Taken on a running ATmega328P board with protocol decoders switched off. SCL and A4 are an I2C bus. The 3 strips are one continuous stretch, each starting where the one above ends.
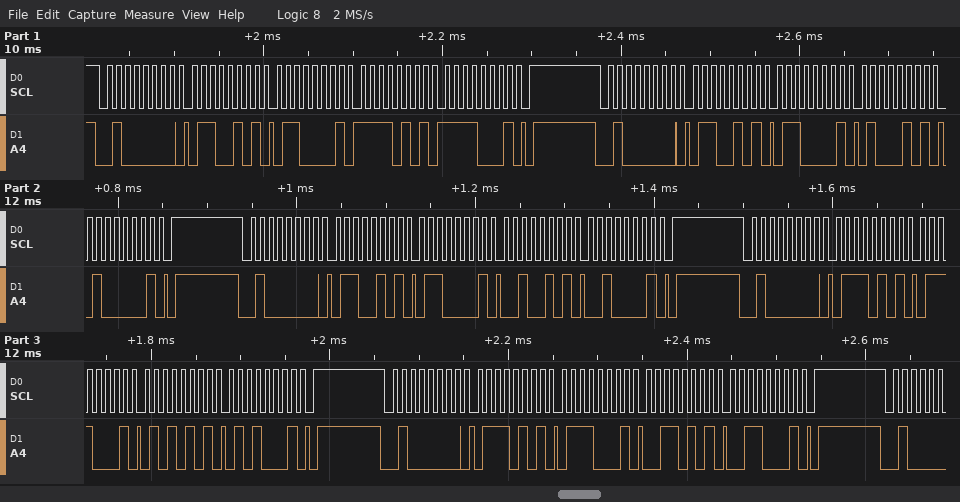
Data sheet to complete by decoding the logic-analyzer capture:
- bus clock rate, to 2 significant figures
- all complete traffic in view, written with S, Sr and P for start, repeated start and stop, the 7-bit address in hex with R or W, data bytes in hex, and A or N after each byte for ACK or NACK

100 kHz
S 20W A 65 A 61 A F5 A F1 A P S 20W A 65 A 61 A 45 A 41 A P S 20W A 65 A 61 A 25 A 21 A P S 20W A 75 A 71 A 55 A 51 A P S 20W A 75 A 71 A 35 A 31 A P
